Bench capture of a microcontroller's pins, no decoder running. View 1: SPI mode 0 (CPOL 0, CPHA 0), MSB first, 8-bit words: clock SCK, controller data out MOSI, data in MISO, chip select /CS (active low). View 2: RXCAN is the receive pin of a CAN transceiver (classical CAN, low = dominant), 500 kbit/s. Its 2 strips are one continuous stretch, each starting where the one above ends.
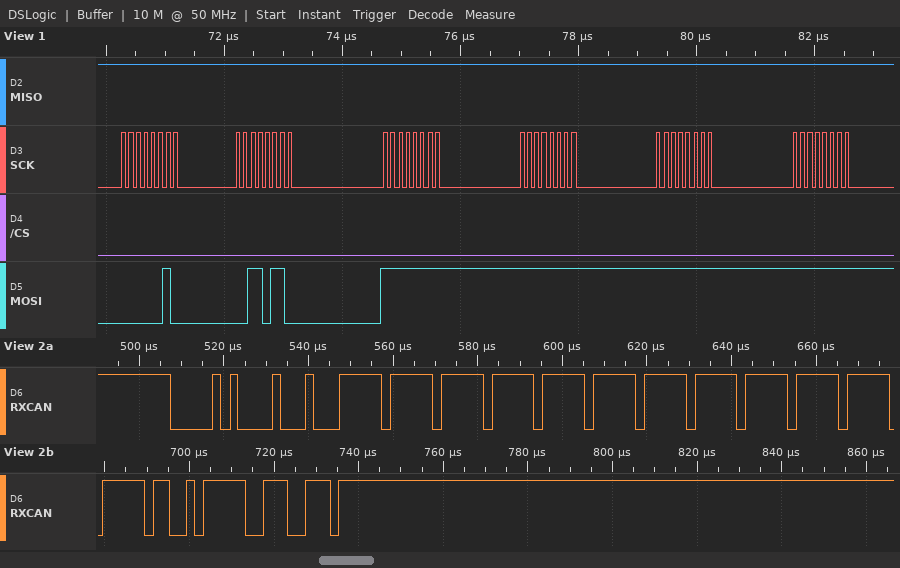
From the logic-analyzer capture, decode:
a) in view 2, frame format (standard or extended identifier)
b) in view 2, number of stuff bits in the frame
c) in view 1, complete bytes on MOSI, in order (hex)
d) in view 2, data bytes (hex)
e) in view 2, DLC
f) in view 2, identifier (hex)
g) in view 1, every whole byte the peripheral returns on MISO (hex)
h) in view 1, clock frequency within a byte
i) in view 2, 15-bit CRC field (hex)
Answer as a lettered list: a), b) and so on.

a) standard
b) 14
c) 0x02 0x36 0xFF 0xFF 0xFF 0xFF
d) FF FF FF FF FF FF FF FC
e) 8
f) 0x021
g) 0xFF 0xFF 0xFF 0xFF 0xFF 0xFF
h) 8 MHz
i) 0x5F73
